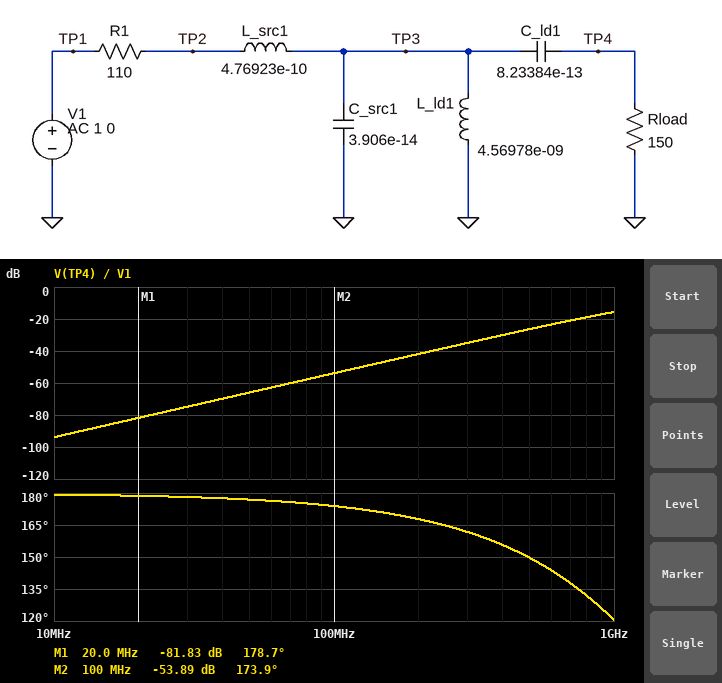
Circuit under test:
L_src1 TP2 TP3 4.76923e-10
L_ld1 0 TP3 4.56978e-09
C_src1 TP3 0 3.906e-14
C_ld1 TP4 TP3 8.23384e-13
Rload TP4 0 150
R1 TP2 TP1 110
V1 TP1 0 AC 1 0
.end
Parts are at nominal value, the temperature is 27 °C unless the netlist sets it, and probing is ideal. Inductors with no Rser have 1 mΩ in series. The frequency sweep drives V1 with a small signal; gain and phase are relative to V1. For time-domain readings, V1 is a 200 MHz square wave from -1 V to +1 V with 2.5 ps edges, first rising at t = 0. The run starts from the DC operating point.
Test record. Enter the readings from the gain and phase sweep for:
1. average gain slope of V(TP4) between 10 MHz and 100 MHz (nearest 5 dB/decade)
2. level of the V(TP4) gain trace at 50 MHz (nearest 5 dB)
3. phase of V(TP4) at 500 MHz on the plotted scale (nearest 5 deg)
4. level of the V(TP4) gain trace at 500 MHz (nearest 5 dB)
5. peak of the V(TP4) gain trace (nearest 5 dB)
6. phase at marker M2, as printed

40 dB/decade
-65 dB
150 deg
-25 dB
-15 dB
173.9 deg
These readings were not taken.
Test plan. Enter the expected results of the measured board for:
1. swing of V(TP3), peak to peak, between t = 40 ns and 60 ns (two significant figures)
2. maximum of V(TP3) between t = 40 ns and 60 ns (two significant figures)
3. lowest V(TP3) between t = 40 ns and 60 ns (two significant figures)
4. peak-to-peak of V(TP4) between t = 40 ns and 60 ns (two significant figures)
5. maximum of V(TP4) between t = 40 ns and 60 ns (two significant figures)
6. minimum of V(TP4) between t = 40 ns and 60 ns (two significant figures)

2.3 V
1.1 V
-1.1 V
2.2 V
1.1 V
-1.1 V
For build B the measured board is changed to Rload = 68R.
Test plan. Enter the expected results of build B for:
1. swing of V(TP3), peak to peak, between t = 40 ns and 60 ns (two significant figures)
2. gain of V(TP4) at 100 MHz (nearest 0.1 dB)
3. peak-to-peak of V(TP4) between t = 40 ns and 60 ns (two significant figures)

1.6 V
-60.7 dB
1.4 V
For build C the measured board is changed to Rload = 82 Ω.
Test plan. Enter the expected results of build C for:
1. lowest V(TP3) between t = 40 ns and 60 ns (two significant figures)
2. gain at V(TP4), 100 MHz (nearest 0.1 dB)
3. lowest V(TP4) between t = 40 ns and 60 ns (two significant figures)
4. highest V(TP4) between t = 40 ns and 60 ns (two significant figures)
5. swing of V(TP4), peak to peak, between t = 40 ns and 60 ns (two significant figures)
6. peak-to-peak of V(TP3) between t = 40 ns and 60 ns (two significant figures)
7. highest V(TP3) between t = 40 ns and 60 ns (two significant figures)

-860 mV
-59.1 dB
-770 mV
770 mV
1.5 V
1.7 V
860 mV
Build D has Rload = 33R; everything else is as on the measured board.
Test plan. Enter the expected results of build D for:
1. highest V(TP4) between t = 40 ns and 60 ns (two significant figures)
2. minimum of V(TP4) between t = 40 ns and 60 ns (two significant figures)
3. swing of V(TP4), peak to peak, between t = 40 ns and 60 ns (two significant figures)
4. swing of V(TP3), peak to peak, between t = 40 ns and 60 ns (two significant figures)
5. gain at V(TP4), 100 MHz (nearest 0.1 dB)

400 mV
-400 mV
800 mV
1.4 V
-67.0 dB
